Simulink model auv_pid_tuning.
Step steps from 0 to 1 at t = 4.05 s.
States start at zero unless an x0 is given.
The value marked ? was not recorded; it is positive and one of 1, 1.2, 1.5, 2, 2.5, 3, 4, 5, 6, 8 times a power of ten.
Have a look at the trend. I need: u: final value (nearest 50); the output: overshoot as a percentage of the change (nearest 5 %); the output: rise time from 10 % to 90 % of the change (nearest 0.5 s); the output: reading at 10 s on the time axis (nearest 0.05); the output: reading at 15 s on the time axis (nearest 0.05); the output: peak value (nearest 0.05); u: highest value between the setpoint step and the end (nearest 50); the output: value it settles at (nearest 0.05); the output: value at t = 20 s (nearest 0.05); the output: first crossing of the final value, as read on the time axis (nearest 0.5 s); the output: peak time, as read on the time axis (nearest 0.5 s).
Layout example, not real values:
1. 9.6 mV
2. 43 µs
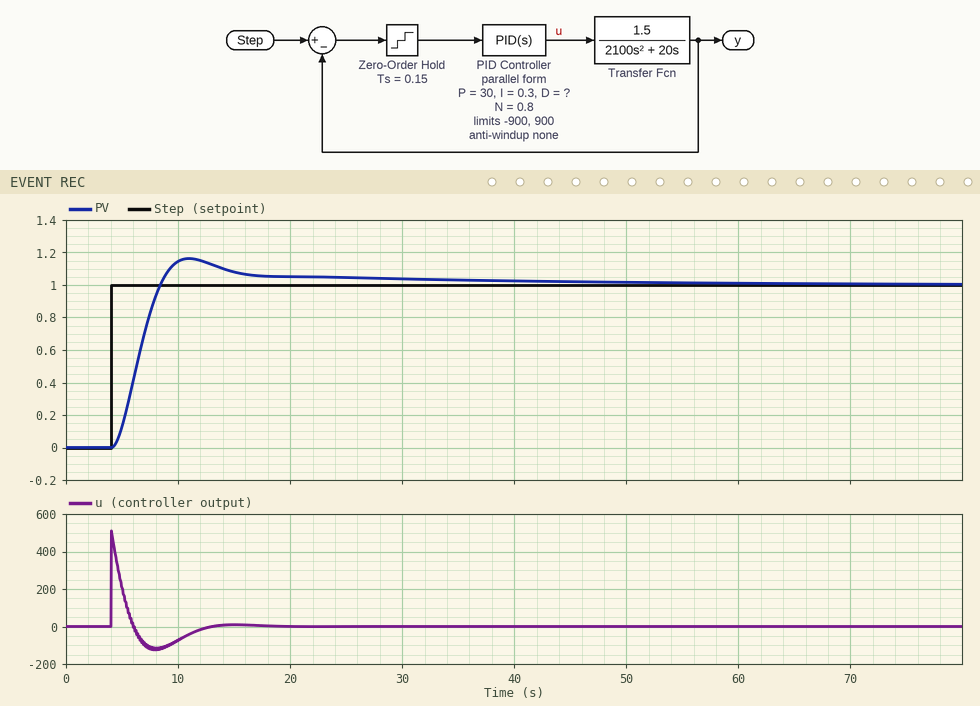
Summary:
1. 0
2. 15 %
3. 3.0 s
4. 1.15
5. 1.10
6. 1.15
7. 500
8. 1.00
9. 1.05
10. 8.5 s
11. 11.0 s
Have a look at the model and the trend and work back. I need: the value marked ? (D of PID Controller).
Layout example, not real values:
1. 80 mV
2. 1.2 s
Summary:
1. 600
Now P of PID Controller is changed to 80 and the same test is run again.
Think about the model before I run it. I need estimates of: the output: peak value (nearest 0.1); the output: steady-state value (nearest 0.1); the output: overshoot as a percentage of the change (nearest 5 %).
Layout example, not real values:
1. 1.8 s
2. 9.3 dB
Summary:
1. 1.3
2. 1.0
3. 30 %
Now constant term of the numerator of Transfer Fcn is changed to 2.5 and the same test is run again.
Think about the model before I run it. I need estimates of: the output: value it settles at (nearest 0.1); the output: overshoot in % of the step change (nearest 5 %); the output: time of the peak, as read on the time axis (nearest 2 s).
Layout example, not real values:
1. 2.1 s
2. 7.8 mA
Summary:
1. 1.0
2. 25 %
3. 8 s
